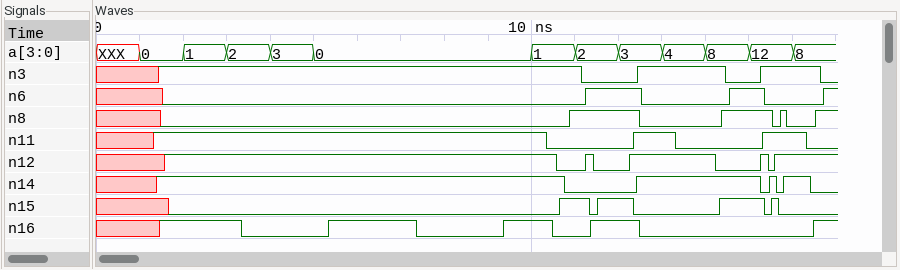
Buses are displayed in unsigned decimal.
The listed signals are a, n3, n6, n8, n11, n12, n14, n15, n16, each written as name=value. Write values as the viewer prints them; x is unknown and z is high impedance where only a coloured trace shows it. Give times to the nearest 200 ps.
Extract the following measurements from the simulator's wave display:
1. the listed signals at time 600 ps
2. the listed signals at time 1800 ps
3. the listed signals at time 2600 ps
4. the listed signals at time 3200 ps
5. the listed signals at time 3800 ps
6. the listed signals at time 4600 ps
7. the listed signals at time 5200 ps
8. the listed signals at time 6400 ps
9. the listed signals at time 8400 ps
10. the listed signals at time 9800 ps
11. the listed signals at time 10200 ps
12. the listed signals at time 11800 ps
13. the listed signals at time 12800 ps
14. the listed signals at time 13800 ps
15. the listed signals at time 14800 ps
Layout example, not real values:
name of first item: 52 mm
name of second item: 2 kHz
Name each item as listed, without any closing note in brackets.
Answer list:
the listed signals at time 600 ps: a=XXX, n3=x, n6=x, n8=x, n11=x, n12=x, n14=x, n15=x, n16=x
the listed signals at time 1800 ps: a=0, n3=1, n6=0, n8=0, n11=1, n12=1, n14=1, n15=0, n16=1
the listed signals at time 2600 ps: a=1, n3=1, n6=0, n8=0, n11=1, n12=1, n14=1, n15=0, n16=1
the listed signals at time 3200 ps: a=2, n3=1, n6=0, n8=0, n11=1, n12=1, n14=1, n15=0, n16=1
the listed signals at time 3800 ps: a=2, n3=1, n6=0, n8=0, n11=1, n12=1, n14=1, n15=0, n16=0
the listed signals at time 4600 ps: a=3, n3=1, n6=0, n8=0, n11=1, n12=1, n14=1, n15=0, n16=0
the listed signals at time 5200 ps: a=0, n3=1, n6=0, n8=0, n11=1, n12=1, n14=1, n15=0, n16=0
the listed signals at time 6400 ps: a=0, n3=1, n6=0, n8=0, n11=1, n12=1, n14=1, n15=0, n16=1
the listed signals at time 8400 ps: a=0, n3=1, n6=0, n8=0, n11=1, n12=1, n14=1, n15=0, n16=0
the listed signals at time 9800 ps: a=0, n3=1, n6=0, n8=0, n11=1, n12=1, n14=1, n15=0, n16=1
the listed signals at time 10200 ps: a=1, n3=1, n6=0, n8=0, n11=1, n12=1, n14=1, n15=0, n16=1
the listed signals at time 11800 ps: a=2, n3=0, n6=1, n8=1, n11=0, n12=0, n14=0, n15=1, n16=1
the listed signals at time 12800 ps: a=3, n3=1, n6=0, n8=0, n11=1, n12=1, n14=1, n15=0, n16=0
the listed signals at time 13800 ps: a=4, n3=1, n6=0, n8=0, n11=0, n12=1, n14=1, n15=0, n16=0
the listed signals at time 14800 ps: a=8, n3=0, n6=1, n8=1, n11=0, n12=0, n14=1, n15=1, n16=0
